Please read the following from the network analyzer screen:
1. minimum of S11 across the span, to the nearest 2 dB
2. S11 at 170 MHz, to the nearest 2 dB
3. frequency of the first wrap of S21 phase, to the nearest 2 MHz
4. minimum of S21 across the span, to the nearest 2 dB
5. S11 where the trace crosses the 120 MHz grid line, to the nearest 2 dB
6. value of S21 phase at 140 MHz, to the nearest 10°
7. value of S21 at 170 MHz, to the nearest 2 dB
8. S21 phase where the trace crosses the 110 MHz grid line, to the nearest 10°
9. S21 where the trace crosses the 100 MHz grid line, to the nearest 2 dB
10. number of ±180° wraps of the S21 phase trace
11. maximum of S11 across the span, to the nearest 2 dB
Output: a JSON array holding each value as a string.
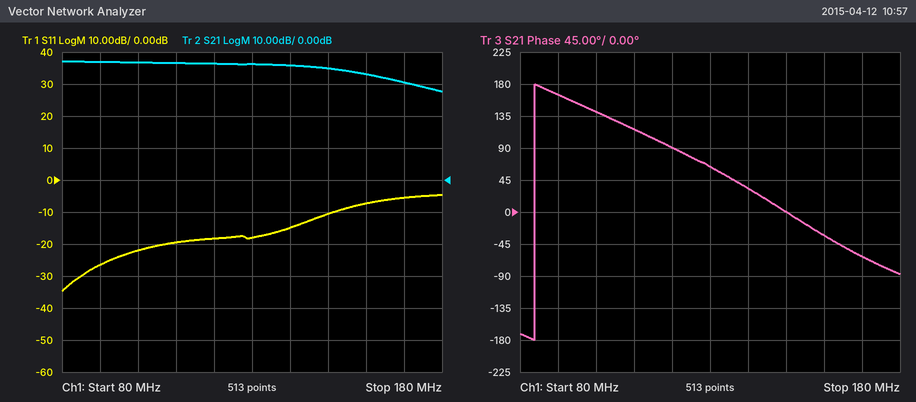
["-34 dB", "-6 dB", "84 MHz", "28 dB", "-18 dB", "30°", "30 dB", "120°", "36 dB", "1", "-4 dB"]
